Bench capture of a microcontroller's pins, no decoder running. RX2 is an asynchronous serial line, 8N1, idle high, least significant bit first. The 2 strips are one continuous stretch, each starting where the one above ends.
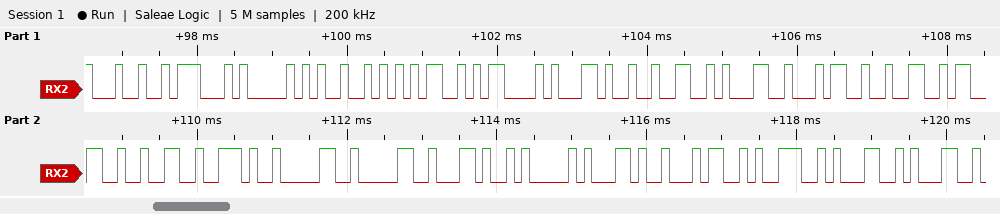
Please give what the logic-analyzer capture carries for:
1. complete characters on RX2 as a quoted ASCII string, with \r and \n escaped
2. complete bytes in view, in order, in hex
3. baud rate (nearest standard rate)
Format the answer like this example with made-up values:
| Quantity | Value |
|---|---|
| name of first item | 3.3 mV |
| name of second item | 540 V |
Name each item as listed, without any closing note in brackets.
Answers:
| Quantity | Value |
|---|---|
| complete characters on RX2 as a quoted ASCII string, with \r and \n escaped | "$GPRMC,214232.00,A,4911" |
| complete bytes in view, in order, in hex | 0x24 0x47 0x50 0x52 0x4D 0x43 0x2C 0x32 0x31 0x34 0x32 0x33 0x32 0x2E 0x30 0x30 0x2C 0x41 0x2C 0x34 0x39 0x31 0x31 |
| baud rate | 9600 baud |
